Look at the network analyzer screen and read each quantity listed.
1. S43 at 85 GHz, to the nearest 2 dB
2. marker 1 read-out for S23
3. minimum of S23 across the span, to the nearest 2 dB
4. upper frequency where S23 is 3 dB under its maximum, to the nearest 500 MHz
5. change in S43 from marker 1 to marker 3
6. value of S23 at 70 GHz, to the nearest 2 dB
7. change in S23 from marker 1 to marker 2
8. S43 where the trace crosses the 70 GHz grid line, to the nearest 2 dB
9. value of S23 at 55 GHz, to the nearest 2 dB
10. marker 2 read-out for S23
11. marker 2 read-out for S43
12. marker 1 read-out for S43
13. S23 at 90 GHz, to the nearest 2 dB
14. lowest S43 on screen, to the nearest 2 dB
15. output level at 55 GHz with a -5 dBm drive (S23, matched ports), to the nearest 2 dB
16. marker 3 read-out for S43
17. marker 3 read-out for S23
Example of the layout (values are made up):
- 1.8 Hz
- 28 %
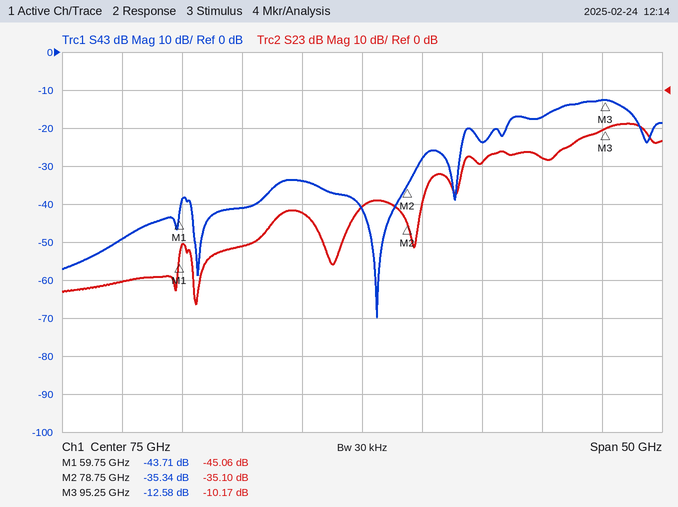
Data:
- -24 dB
- -45.06 dB
- -56 dB
- 99.0 GHz
- 31.13 dB
- -32 dB
- 9.96 dB
- -34 dB
- -50 dB
- -35.10 dB
- -35.34 dB
- -43.71 dB
- -18 dB
- -70 dB
- -56 dBm
- -12.58 dB
- -10.17 dB
